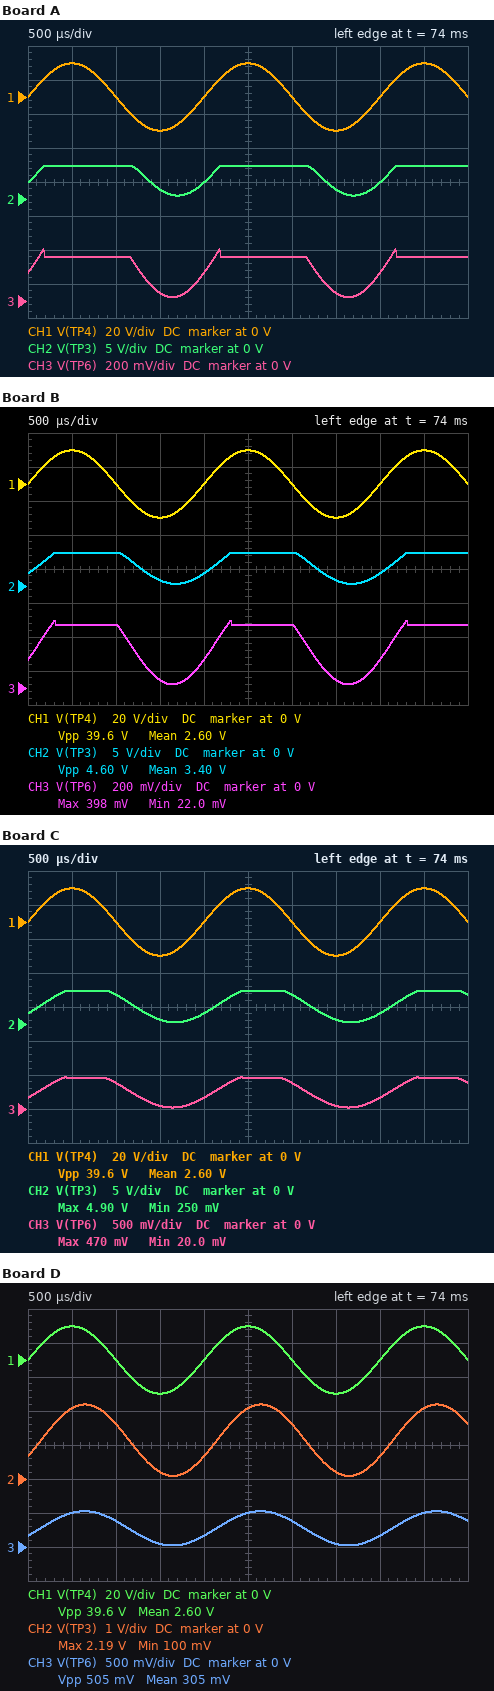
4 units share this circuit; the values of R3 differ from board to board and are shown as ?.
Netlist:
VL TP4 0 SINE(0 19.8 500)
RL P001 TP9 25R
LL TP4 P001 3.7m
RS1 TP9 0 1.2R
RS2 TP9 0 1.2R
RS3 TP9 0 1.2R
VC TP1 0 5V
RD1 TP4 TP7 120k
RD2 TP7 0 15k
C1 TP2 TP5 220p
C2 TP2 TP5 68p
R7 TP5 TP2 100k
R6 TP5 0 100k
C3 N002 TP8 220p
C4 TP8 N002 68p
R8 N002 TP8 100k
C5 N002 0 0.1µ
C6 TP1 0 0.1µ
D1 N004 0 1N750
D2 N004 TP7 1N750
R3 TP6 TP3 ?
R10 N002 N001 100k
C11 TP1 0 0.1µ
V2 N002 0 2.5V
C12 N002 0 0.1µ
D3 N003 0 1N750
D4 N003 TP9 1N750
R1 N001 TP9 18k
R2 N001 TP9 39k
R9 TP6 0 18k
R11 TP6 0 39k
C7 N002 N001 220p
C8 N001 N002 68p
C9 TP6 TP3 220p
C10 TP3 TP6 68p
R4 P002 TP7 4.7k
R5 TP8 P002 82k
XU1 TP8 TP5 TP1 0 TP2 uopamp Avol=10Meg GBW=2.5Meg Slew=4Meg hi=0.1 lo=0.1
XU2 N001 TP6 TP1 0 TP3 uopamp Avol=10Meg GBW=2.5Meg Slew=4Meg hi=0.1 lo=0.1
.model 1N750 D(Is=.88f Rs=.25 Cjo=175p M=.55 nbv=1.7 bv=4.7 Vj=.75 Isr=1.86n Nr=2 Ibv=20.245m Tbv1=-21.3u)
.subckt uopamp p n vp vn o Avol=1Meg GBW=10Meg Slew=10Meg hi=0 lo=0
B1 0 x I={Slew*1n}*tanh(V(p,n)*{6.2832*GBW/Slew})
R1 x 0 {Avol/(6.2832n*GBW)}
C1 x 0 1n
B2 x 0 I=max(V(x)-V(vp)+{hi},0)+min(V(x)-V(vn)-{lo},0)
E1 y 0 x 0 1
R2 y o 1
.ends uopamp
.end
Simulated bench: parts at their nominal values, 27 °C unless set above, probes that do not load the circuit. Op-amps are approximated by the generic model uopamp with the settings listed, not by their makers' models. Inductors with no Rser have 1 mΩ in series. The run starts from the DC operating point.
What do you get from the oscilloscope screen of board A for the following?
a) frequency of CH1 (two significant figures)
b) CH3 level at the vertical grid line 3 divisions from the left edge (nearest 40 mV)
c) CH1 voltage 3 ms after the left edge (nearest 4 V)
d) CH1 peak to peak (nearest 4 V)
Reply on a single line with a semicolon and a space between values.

500 Hz; 40 mV; 0 V; 40 V
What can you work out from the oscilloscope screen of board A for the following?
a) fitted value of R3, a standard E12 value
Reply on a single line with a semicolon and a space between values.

220 kΩ
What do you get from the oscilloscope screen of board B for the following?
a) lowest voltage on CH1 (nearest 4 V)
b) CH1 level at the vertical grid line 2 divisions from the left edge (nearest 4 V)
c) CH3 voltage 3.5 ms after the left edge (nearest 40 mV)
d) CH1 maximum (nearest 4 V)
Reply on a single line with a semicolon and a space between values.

-20 V; 0 V; 40 mV; 20 V
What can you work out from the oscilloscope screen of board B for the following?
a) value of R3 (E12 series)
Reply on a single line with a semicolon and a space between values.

150 kΩ
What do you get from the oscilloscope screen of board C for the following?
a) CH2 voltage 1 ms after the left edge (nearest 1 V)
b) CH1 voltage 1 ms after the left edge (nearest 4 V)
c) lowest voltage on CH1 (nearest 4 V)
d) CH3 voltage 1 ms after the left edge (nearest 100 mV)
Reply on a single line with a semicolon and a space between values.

4 V; 0 V; -20 V; 400 mV
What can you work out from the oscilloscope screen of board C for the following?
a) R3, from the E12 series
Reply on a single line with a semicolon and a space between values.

120 kΩ
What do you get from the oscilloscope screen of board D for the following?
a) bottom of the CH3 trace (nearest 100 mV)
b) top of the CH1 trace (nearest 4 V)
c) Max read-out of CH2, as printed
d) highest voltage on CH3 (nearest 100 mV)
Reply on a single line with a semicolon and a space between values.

0 V; 20 V; 2.19 V; 500 mV
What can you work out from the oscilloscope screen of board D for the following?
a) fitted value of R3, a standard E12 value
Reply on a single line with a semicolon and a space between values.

39 kΩ
